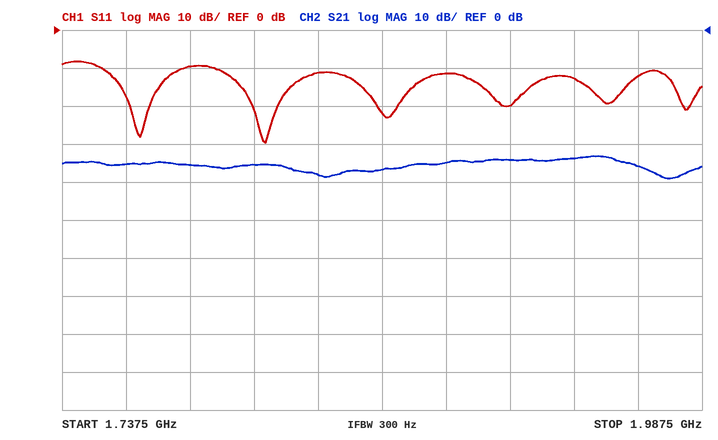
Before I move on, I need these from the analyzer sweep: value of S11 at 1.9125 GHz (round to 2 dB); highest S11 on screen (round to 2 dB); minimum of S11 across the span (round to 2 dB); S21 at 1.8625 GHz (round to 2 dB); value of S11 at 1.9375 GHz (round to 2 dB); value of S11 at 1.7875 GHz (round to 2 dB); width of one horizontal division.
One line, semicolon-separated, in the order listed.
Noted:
-20 dB; -8 dB; -30 dB; -36 dB; -12 dB; -10 dB; 25 MHz
